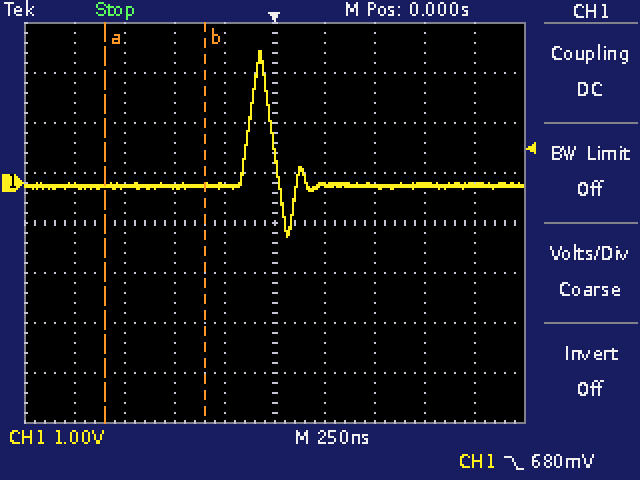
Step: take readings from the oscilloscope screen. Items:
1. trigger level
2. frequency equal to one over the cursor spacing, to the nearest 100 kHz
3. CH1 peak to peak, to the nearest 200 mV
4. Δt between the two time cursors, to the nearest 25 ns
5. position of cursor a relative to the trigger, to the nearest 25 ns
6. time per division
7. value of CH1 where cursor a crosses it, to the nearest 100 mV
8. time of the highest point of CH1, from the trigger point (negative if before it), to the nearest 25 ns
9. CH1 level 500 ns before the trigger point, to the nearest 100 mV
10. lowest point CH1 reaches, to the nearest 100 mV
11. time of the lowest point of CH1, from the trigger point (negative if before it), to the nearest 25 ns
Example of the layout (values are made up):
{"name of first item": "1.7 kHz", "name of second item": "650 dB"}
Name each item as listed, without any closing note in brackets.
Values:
{"trigger level": "680 mV", "frequency equal to one over the cursor spacing, to the nearest 100 kHz": "2.0 MHz", "CH1 peak to peak, to the nearest 200 mV": "3.8 V", "Δt between the two time cursors, to the nearest 25 ns": "500 ns", "position of cursor a relative to the trigger, to the nearest 25 ns": "-850 ns", "time per division": "250 ns", "value of CH1 where cursor a crosses it, to the nearest 100 mV": "-100 mV", "time of the highest point of CH1, from the trigger point (negative if before it), to the nearest 25 ns": "-75 ns", "CH1 level 500 ns before the trigger point, to the nearest 100 mV": "-100 mV", "lowest point CH1 reaches, to the nearest 100 mV": "-1.1 V", "time of the lowest point of CH1, from the trigger point (negative if before it), to the nearest 25 ns": "+75 ns"}
